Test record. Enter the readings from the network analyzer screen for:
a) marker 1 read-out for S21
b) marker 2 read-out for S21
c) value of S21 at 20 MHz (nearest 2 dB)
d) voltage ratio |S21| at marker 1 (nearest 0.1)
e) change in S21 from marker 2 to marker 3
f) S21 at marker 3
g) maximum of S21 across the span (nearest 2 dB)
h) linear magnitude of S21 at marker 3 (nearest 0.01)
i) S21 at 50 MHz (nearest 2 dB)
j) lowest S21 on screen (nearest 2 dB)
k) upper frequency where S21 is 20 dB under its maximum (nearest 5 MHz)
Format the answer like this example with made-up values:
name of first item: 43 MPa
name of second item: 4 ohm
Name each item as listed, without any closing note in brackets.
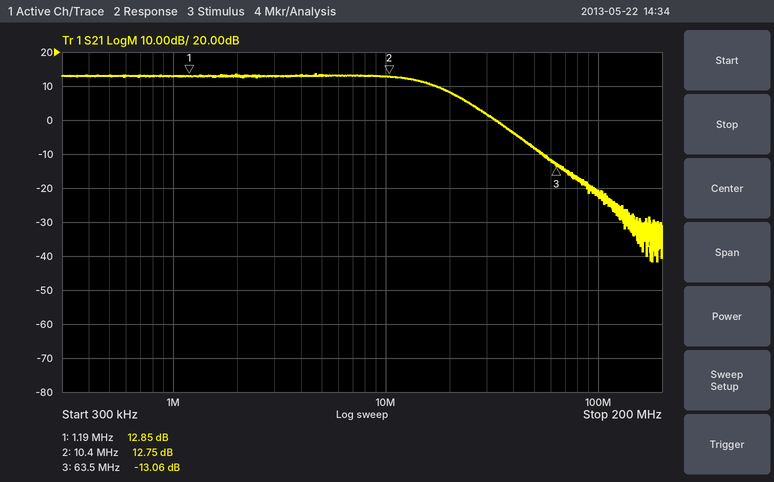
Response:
marker 1 read-out for S21: 12.85 dB
marker 2 read-out for S21: 12.75 dB
value of S21 at 20 MHz: 8 dB
voltage ratio |S21| at marker 1: 4.4
change in S21 from marker 2 to marker 3: -25.81 dB
S21 at marker 3: -13.06 dB
maximum of S21 across the span: 14 dB
linear magnitude of S21 at marker 3: 0.22
S21 at 50 MHz: -8 dB
lowest S21 on screen: -42 dB
upper frequency where S21 is 20 dB under its maximum: 45 MHz
